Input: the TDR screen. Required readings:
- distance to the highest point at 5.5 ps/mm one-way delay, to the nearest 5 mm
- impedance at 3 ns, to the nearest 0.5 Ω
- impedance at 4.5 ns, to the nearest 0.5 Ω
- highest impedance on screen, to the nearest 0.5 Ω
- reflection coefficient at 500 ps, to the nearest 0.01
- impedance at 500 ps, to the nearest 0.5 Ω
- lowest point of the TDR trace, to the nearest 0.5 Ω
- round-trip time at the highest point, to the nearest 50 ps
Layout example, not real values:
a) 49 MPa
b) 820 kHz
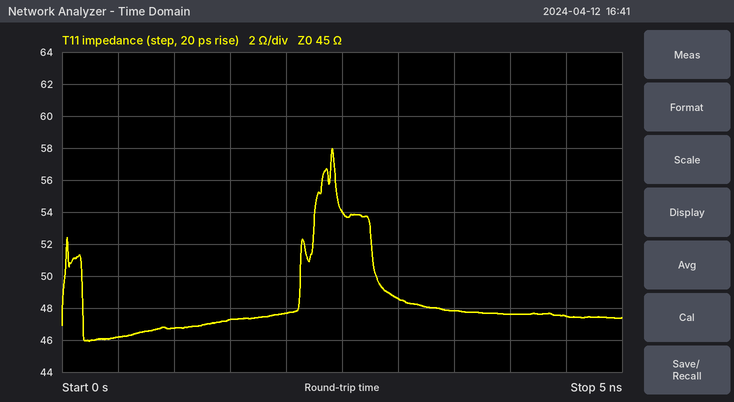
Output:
a) 220 mm
b) 48.5 Ω
c) 47.5 Ω
d) 58.0 Ω
e) +0.01
f) 46.0 Ω
g) 46.0 Ω
h) 2.40 ns
